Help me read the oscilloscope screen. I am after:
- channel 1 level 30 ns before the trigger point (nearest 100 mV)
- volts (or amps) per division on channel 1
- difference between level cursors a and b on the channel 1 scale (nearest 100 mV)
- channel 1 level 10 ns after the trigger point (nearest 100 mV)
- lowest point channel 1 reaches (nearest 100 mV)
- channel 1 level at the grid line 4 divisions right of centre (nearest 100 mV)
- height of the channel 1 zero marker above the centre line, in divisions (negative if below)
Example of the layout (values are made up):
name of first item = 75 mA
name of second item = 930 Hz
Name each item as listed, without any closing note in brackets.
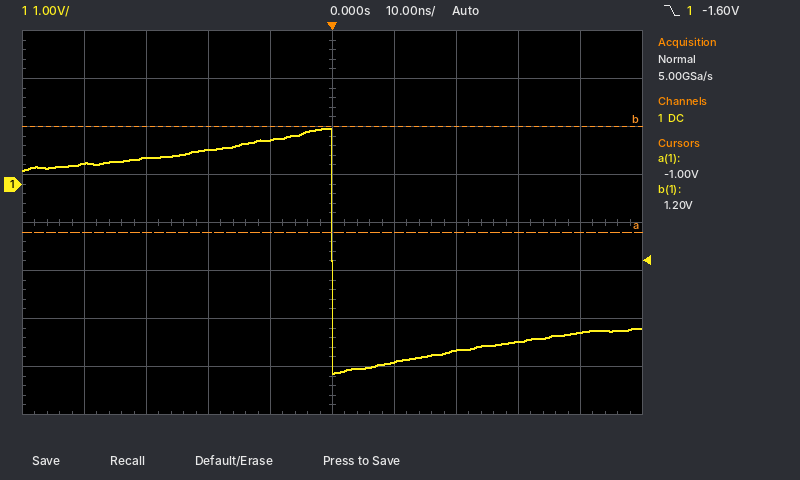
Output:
channel 1 level 30 ns before the trigger point = 600 mV
volts (or amps) per division on channel 1 = 1 V
difference between level cursors a and b on the channel 1 scale = 2.2 V
channel 1 level 10 ns after the trigger point = -3.7 V
lowest point channel 1 reaches = -3.9 V
channel 1 level at the grid line 4 divisions right of centre = -3.1 V
height of the channel 1 zero marker above the centre line, in divisions = +0.8 div
